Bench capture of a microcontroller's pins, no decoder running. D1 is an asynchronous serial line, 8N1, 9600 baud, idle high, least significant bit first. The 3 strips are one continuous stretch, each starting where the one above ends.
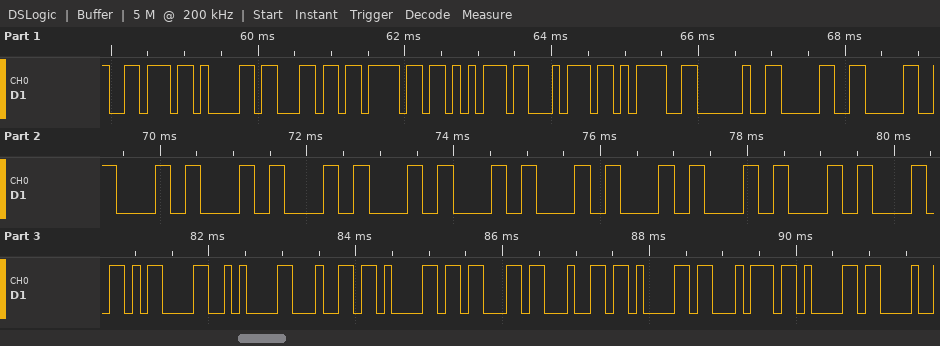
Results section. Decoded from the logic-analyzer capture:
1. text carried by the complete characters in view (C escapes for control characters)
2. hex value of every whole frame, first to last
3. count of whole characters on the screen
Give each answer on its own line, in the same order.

"valout= 000000000000\r\ndacdata"
76 61 6C 6F 75 74 3D 20 30 30 30 30 30 30 30 30 30 30 30 30 0D 0A 64 61 63 64 61 74 61
29
